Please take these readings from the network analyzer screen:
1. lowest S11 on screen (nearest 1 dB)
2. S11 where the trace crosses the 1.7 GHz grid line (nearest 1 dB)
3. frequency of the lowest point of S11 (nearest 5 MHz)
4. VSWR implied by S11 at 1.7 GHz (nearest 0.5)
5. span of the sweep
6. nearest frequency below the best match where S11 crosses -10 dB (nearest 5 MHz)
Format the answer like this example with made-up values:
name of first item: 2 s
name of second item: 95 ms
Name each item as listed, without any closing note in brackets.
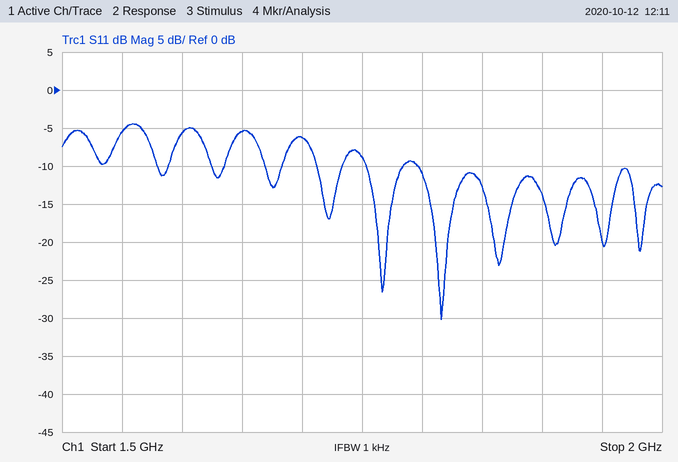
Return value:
lowest S11 on screen: -30 dB
S11 where the trace crosses the 1.7 GHz grid line: -6 dB
frequency of the lowest point of S11: 1.815 GHz
VSWR implied by S11 at 1.7 GHz: 3.0
span of the sweep: 500 MHz
nearest frequency below the best match where S11 crosses -10 dB: 1.795 GHz
